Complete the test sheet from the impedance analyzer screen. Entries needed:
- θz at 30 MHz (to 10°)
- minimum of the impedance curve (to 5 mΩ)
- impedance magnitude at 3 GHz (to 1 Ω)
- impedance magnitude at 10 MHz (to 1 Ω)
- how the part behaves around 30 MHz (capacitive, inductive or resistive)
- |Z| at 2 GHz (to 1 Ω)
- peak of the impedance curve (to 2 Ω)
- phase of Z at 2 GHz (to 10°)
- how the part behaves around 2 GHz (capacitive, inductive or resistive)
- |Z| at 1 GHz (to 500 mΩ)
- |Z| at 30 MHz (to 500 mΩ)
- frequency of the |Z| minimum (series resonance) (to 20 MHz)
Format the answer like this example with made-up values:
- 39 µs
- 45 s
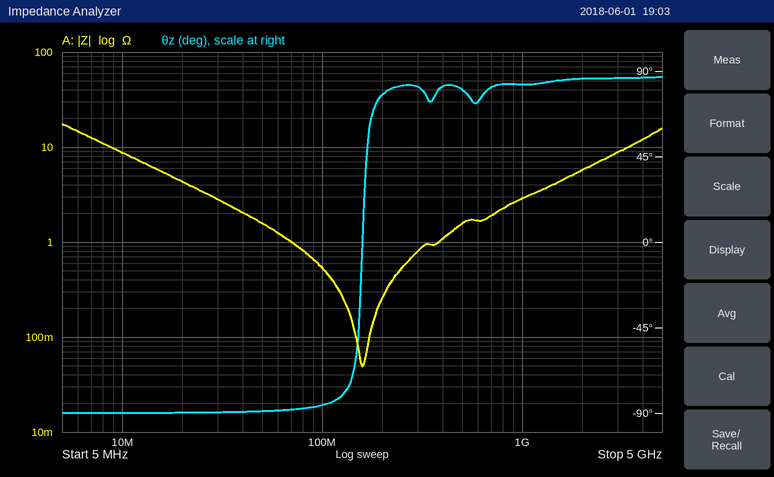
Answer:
- -90°
- 50 mΩ
- 9 Ω
- 9 Ω
- capacitive
- 6 Ω
- 18 Ω
- 90°
- inductive
- 3.0 Ω
- 3.0 Ω
- 160 MHz
